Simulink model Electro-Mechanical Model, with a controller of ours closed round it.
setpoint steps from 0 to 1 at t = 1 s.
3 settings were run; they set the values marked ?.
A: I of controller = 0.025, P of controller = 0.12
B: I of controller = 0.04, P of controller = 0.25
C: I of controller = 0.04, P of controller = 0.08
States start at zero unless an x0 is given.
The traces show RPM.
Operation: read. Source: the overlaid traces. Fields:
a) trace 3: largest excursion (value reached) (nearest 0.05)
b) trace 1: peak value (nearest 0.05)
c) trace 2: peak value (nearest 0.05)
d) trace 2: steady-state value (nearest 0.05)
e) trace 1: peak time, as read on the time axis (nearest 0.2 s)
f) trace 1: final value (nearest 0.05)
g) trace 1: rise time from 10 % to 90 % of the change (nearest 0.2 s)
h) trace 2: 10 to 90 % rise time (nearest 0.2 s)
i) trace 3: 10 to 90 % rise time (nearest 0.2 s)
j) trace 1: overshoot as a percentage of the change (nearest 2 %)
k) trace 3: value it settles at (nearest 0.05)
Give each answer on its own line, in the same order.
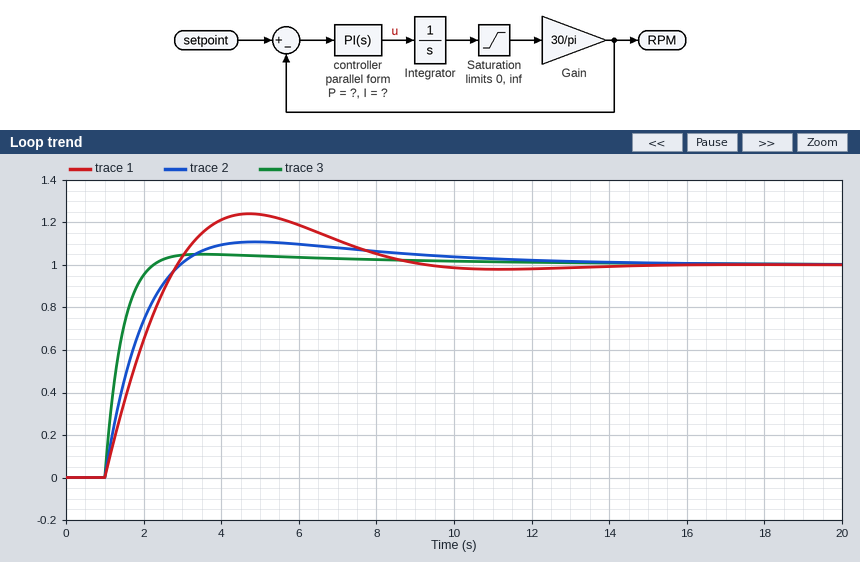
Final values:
1.05
1.25
1.10
1.00
4.8 s
1.00
1.4 s
1.4 s
0.8 s
24 %
1.00
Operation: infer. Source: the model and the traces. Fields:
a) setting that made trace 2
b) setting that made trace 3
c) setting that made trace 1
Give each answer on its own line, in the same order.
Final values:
A
B
C
